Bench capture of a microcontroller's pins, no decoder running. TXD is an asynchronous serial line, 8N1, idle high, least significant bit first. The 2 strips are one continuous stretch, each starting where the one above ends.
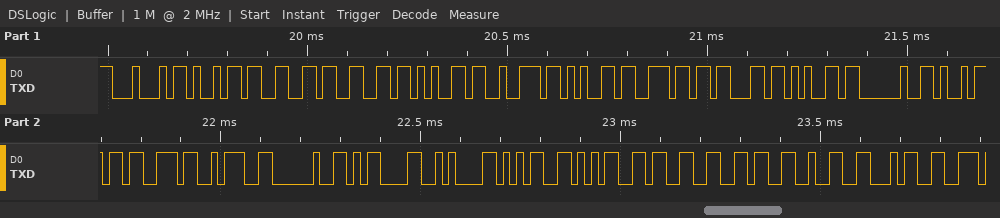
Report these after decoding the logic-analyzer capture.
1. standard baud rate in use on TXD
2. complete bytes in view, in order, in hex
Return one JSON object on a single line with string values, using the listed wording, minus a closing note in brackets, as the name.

{"standard baud rate in use on TXD": "57600 baud", "complete bytes in view, in order, in hex": "44 69 66 66 65 72 65 6E 63 65 20 69 73 3A 20 0D 0A 35 35 33 36 32 34"}
